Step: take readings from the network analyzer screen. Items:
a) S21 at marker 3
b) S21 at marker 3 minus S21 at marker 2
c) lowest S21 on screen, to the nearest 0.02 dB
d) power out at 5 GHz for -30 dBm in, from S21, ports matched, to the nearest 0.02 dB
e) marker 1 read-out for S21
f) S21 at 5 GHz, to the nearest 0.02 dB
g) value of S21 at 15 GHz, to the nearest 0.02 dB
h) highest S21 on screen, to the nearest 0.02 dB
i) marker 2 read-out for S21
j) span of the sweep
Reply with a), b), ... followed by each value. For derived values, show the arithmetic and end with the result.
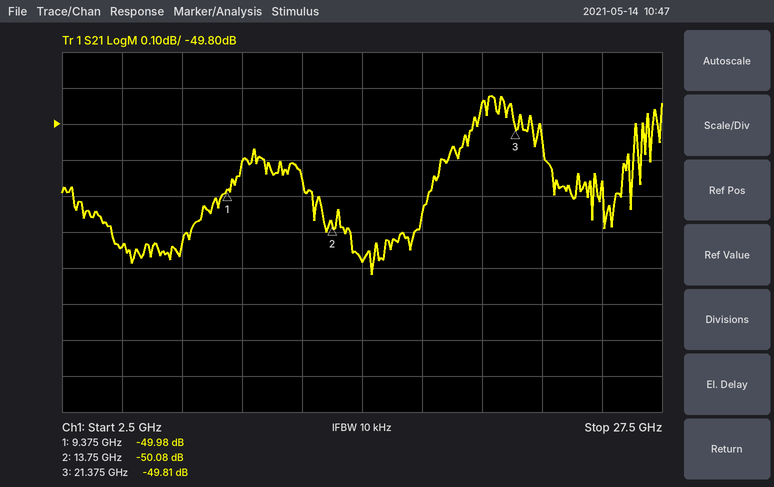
a) -49.81 dB
b) -49.81 − (-50.08) = 0.27 dB
c) -50.22 dB
d) -30 dBm + (-50.14 dB) = -80.14 dBm
e) -49.98 dB
f) -50.14 dB
g) -50.18 dB
h) -49.72 dB
i) -50.08 dB
j) 25 GHz
